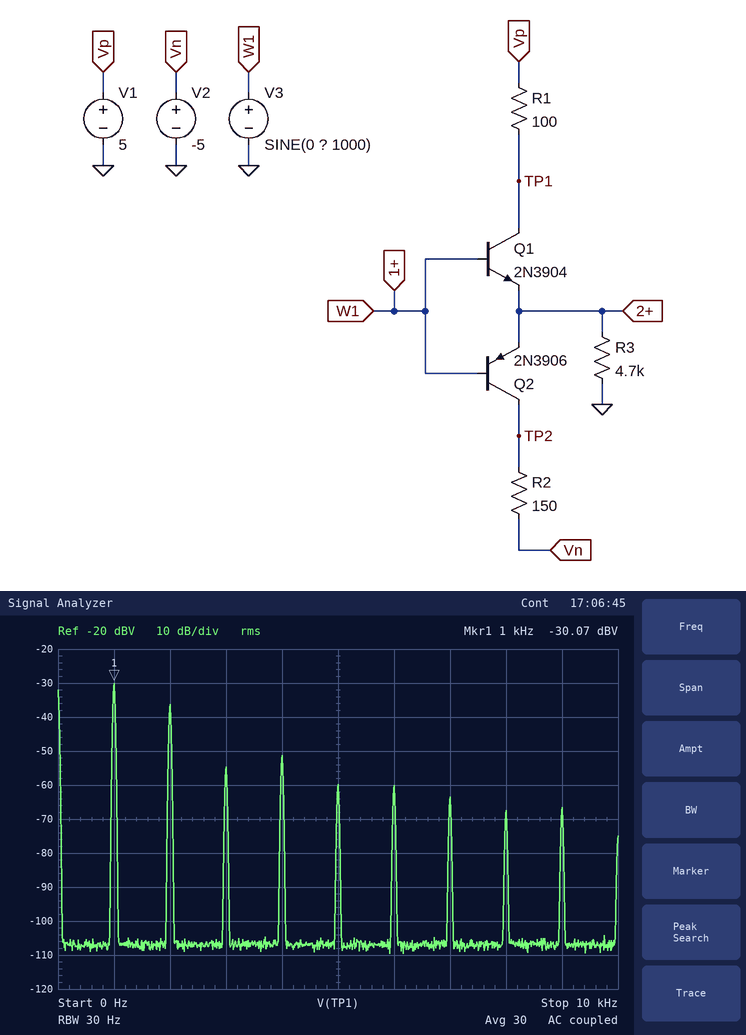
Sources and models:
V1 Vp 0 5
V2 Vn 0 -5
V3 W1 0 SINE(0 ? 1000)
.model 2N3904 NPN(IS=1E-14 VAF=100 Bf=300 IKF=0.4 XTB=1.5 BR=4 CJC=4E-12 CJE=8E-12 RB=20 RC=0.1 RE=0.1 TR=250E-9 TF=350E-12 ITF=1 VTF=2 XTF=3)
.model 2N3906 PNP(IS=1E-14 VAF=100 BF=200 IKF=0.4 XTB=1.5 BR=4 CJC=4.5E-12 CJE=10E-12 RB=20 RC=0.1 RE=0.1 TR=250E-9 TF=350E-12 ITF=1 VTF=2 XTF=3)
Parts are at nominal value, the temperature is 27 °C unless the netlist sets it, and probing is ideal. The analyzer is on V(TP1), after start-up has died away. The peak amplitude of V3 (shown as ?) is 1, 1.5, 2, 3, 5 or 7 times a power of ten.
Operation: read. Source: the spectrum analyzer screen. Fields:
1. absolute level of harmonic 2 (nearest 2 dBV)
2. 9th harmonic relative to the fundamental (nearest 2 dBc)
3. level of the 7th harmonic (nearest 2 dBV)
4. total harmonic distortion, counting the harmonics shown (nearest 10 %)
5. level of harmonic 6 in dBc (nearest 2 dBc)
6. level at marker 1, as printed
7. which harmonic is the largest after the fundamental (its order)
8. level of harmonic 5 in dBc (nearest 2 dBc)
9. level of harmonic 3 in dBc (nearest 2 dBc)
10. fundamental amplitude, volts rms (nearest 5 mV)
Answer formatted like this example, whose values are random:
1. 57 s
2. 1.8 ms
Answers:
1. -36 dBV
2. -36 dBc
3. -64 dBV
4. 50 %
5. -30 dBc
6. -30.07 dBV
7. 2
8. -30 dBc
9. -24 dBc
10. 30 mV
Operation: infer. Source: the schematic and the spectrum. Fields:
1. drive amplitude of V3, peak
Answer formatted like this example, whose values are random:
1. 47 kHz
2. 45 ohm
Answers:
1. 5 V
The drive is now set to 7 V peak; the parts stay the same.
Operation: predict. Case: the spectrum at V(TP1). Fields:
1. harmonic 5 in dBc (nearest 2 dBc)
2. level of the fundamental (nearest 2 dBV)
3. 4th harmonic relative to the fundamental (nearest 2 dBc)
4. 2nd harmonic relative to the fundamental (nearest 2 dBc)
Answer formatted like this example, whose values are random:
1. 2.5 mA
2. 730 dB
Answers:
1. -8 dBc
2. -16 dBV
3. -4 dBc
4. 0 dBc
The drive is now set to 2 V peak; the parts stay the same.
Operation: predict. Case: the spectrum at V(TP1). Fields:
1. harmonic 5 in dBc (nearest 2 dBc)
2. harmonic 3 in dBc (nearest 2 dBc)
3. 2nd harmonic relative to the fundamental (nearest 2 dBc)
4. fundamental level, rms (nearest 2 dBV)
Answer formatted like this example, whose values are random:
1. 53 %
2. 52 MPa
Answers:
1. -22 dBc
2. -16 dBc
3. -4 dBc
4. -40 dBV
